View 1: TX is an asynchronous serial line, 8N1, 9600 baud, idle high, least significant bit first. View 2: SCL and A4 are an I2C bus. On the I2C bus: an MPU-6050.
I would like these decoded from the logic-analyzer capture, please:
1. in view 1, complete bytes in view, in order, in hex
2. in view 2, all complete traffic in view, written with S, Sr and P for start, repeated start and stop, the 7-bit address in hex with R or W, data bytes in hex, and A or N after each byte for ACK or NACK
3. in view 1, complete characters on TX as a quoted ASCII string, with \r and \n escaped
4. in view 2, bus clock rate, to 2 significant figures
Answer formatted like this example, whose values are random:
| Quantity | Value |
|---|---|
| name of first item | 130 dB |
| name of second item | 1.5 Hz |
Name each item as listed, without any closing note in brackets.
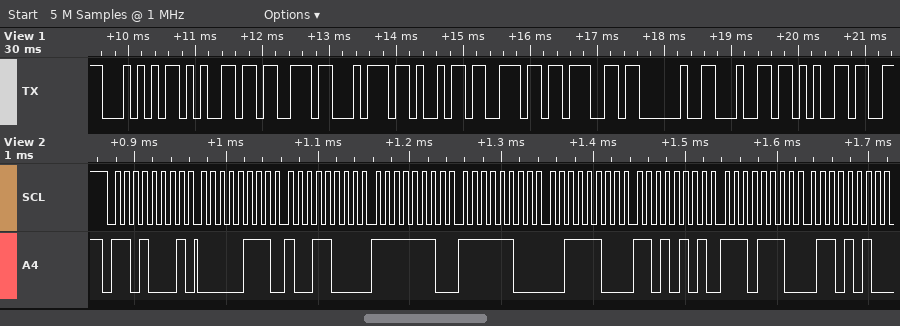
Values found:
| Quantity | Value |
|---|---|
| in view 1, complete bytes in view, in order, in hex | 54 65 73 74 69 6E 67 20 64 65 |
| in view 2, all complete traffic in view, written with S, Sr and P for start, repeated start and stop, the 7-bit address in hex with R or W, data bytes in hex, and A or N after each byte for ACK or NACK | S 68R A 07 A 98 A FE A FC A 3C A D5 A EE A 6A A |
| in view 1, complete characters on TX as a quoted ASCII string, with \r and \n escaped | "Testing de" |
| in view 2, bus clock rate, to 2 significant figures | 100 kHz |
